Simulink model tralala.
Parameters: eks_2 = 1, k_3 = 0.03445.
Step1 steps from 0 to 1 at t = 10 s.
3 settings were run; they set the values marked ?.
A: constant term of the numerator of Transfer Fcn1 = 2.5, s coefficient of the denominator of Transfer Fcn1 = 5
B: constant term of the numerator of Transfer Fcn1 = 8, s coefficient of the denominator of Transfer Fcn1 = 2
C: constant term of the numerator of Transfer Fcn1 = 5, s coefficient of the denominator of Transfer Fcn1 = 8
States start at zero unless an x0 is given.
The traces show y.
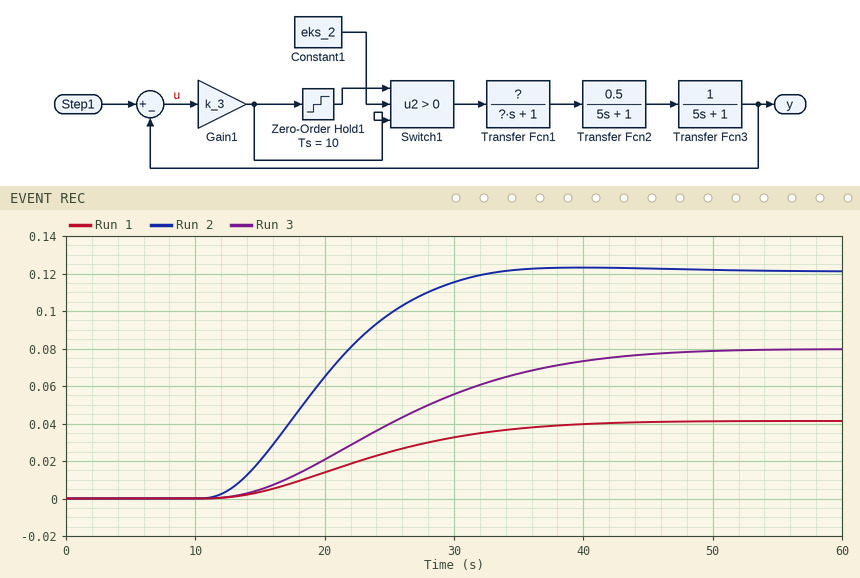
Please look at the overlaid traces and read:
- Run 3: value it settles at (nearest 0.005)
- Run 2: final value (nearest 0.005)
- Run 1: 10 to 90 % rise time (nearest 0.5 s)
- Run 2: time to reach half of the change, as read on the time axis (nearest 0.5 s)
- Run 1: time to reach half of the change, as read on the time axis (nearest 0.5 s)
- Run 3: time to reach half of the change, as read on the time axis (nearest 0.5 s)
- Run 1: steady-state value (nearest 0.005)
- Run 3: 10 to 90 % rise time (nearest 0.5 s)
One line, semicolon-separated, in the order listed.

0.080; 0.120; 19.5 s; 19.5 s; 23.0 s; 25.0 s; 0.040; 22.0 s
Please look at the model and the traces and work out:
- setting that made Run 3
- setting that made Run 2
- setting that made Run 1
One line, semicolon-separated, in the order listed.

C; B; A
